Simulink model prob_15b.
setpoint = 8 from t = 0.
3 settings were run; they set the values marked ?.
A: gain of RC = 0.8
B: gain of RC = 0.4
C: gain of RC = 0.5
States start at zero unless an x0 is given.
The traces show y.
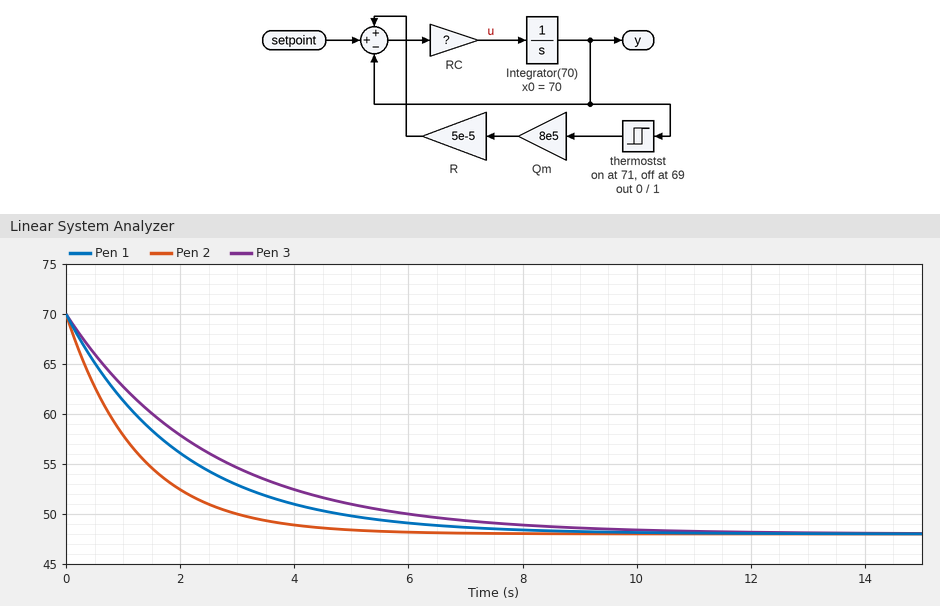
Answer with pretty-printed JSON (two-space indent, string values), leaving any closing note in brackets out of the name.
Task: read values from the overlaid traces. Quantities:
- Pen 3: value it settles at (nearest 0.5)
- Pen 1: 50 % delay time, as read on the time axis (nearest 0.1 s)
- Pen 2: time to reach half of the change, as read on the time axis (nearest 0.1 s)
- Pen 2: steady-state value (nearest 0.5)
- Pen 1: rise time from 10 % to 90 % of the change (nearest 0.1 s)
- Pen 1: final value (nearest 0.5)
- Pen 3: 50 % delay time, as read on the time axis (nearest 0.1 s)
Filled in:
{
  "Pen 3: value it settles at": "48.0",
  "Pen 1: 50 % delay time, as read on the time axis": "1.4 s",
  "Pen 2: time to reach half of the change, as read on the time axis": "0.9 s",
  "Pen 2: steady-state value": "48.0",
  "Pen 1: rise time from 10 % to 90 % of the change": "4.4 s",
  "Pen 1: final value": "48.0",
  "Pen 3: 50 % delay time, as read on the time axis": "1.7 s"
}
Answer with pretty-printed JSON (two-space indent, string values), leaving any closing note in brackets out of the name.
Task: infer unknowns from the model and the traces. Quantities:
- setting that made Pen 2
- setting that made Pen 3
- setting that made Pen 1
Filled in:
{
  "setting that made Pen 2": "A",
  "setting that made Pen 3": "B",
  "setting that made Pen 1": "C"
}
